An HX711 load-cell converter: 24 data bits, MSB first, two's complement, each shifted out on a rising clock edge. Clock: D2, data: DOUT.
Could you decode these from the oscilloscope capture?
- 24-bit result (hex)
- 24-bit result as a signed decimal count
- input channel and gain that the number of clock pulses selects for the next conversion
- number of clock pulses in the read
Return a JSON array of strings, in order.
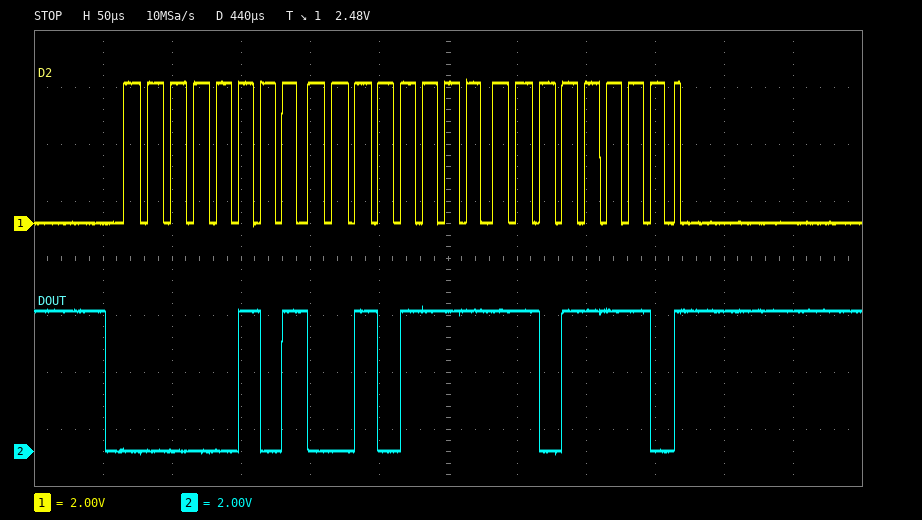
["0x052FDE", "339934", "channel A, gain 128", "25"]
